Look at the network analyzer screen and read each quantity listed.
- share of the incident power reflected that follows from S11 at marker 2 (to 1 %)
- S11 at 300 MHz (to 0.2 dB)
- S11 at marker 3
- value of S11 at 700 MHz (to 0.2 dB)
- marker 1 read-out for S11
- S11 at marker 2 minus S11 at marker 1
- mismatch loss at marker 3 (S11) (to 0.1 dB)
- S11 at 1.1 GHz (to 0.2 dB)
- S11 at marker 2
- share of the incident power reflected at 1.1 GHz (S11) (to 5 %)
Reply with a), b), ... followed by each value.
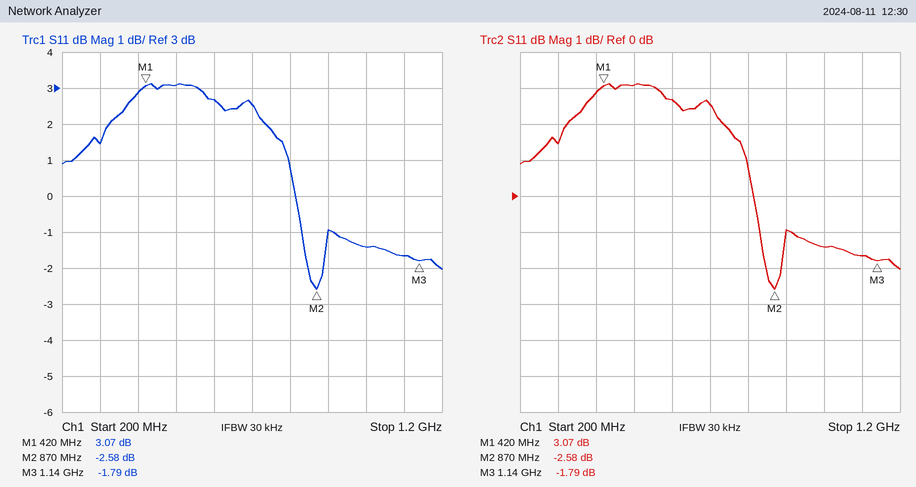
a) 55 %
b) 1.4 dB
c) -1.79 dB
d) 2.6 dB
e) 3.07 dB
f) -5.65 dB
g) 4.7 dB
h) -1.6 dB
i) -2.58 dB
j) 70 %
